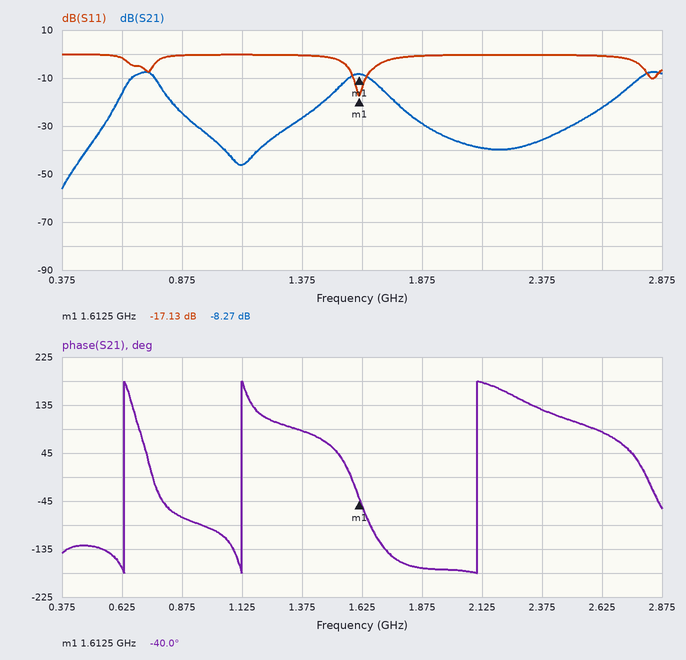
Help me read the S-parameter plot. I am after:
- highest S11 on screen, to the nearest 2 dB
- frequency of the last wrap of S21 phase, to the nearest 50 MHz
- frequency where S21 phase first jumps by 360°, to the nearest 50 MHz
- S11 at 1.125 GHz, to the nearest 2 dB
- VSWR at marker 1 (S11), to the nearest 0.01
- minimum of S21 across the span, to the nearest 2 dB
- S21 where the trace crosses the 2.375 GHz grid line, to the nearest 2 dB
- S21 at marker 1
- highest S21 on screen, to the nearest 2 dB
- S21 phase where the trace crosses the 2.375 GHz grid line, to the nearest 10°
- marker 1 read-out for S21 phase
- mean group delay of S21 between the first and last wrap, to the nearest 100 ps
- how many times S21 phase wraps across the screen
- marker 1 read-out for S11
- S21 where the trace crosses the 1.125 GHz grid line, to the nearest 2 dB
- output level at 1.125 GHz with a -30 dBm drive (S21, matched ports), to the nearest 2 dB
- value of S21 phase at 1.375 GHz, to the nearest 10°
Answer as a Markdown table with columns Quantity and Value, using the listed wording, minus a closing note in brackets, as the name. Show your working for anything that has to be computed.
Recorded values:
| Quantity | Value |
|---|---|
| highest S11 on screen, to the nearest 2 dB | 0 dB |
| frequency of the last wrap of S21 phase, to the nearest 50 MHz | 2.10 GHz |
| frequency where S21 phase first jumps by 360°, to the nearest 50 MHz | 650 MHz |
| S11 at 1.125 GHz, to the nearest 2 dB | 0 dB |
| VSWR at marker 1 (S11), to the nearest 0.01 | (1 + 0.1392)/(1 − 0.1392) ≈ 1.32 |
| minimum of S21 across the span, to the nearest 2 dB | -56 dB |
| S21 where the trace crosses the 2.375 GHz grid line, to the nearest 2 dB | -36 dB |
| S21 at marker 1 | -8.27 dB |
| highest S21 on screen, to the nearest 2 dB | -8 dB |
| S21 phase where the trace crosses the 2.375 GHz grid line, to the nearest 10° | 130° |
| marker 1 read-out for S21 phase | -40.0° |
| mean group delay of S21 between the first and last wrap, to the nearest 100 ps | 2 cycles / (2.10 GHz − 650 MHz) ≈ 1.4 ns |
| how many times S21 phase wraps across the screen | 3 |
| marker 1 read-out for S11 | -17.13 dB |
| S21 where the trace crosses the 1.125 GHz grid line, to the nearest 2 dB | -46 dB |
| output level at 1.125 GHz with a -30 dBm drive (S21, matched ports), to the nearest 2 dB | -30 dBm + (-46 dB) = -76 dBm |
| value of S21 phase at 1.375 GHz, to the nearest 10° | 90° |
